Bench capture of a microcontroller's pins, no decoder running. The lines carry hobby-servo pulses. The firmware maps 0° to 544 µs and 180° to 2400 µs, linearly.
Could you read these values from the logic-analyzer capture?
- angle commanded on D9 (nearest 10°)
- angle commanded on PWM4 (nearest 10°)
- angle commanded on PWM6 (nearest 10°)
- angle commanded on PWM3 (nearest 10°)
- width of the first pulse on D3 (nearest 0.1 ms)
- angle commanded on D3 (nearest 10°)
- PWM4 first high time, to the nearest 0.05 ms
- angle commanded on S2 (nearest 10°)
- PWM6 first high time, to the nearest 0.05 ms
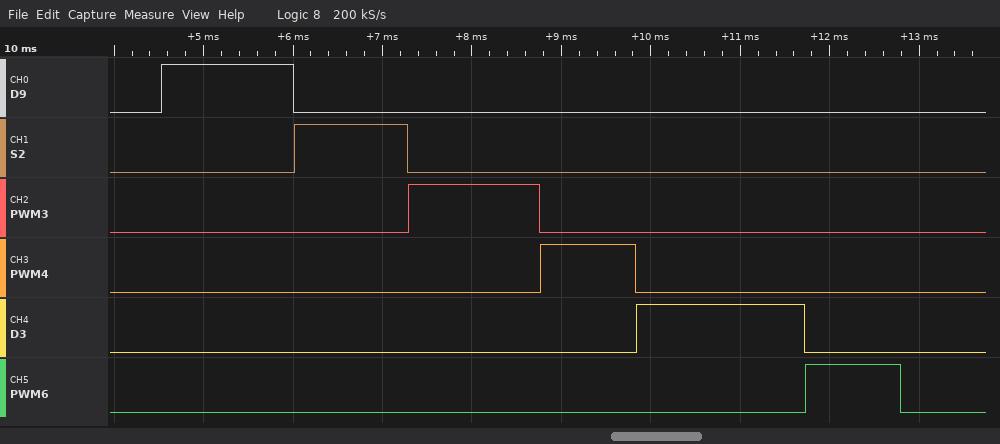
90°
50°
50°
90°
1.9 ms
130°
1.05 ms
70°
1.05 ms
